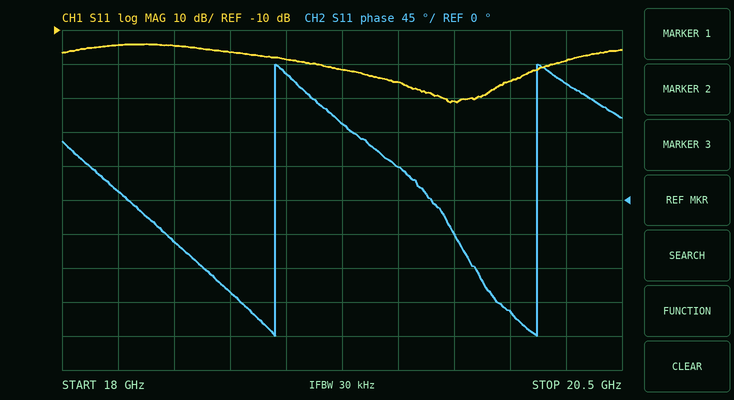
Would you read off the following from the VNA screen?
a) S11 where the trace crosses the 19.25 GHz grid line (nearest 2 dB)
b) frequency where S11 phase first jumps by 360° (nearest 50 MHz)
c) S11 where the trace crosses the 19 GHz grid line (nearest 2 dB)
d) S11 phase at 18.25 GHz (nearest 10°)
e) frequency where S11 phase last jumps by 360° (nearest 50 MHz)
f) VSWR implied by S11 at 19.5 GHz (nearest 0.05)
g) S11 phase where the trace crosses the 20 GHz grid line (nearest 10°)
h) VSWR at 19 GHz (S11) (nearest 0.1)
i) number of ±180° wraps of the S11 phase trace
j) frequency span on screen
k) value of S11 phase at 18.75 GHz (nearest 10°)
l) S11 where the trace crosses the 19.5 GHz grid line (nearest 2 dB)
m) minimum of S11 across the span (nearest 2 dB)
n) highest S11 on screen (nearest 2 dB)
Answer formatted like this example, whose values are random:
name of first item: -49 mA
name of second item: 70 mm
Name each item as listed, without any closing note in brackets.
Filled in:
S11 where the trace crosses the 19.25 GHz grid line: -22 dB
frequency where S11 phase first jumps by 360°: 18.95 GHz
S11 where the trace crosses the 19 GHz grid line: -18 dB
S11 phase at 18.25 GHz: 10°
frequency where S11 phase last jumps by 360°: 20.10 GHz
VSWR implied by S11 at 19.5 GHz: 1.10
S11 phase where the trace crosses the 20 GHz grid line: -150°
VSWR at 19 GHz (S11): 1.3
number of ±180° wraps of the S11 phase trace: 2
frequency span on screen: 2.5 GHz
value of S11 phase at 18.75 GHz: -120°
S11 where the trace crosses the 19.5 GHz grid line: -26 dB
minimum of S11 across the span: -32 dB
highest S11 on screen: -14 dB
